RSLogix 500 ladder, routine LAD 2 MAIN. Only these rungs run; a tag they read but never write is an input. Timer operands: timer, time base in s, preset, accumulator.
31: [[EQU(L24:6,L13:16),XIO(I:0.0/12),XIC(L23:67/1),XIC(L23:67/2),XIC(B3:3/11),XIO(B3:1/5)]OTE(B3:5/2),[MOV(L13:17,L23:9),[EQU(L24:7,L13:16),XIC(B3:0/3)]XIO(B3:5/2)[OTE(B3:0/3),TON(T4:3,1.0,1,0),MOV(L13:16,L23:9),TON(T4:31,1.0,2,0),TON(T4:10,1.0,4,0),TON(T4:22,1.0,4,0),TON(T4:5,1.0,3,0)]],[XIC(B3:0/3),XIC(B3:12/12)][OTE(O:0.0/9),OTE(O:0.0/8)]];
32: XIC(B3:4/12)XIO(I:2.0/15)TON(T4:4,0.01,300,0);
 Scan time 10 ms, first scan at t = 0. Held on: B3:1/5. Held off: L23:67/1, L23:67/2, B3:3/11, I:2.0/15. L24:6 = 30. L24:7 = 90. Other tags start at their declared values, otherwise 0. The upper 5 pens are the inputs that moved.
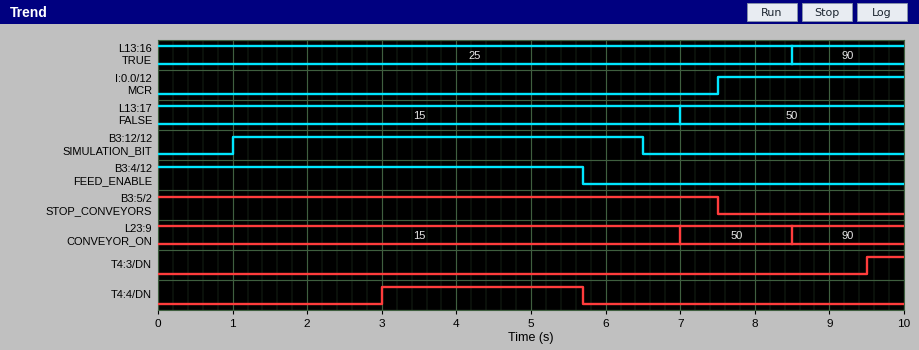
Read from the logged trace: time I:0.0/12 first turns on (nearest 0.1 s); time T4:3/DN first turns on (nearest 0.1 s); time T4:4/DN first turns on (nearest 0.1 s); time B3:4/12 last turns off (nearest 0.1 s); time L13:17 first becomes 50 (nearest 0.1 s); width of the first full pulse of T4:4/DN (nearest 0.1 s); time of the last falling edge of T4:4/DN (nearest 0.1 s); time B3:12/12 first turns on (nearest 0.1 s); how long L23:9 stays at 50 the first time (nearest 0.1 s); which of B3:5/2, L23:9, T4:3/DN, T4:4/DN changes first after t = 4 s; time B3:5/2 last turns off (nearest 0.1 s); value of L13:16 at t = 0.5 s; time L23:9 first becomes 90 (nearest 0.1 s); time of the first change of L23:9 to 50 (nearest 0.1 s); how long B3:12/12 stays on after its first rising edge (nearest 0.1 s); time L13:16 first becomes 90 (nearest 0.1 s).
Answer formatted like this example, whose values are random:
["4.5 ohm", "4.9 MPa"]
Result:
["7.5 s", "9.5 s", "3.0 s", "5.7 s", "7.0 s", "2.7 s", "5.7 s", "1.0 s", "1.5 s", "T4:4/DN", "7.5 s", "25", "8.5 s", "7.0 s", "5.5 s", "8.5 s"]
